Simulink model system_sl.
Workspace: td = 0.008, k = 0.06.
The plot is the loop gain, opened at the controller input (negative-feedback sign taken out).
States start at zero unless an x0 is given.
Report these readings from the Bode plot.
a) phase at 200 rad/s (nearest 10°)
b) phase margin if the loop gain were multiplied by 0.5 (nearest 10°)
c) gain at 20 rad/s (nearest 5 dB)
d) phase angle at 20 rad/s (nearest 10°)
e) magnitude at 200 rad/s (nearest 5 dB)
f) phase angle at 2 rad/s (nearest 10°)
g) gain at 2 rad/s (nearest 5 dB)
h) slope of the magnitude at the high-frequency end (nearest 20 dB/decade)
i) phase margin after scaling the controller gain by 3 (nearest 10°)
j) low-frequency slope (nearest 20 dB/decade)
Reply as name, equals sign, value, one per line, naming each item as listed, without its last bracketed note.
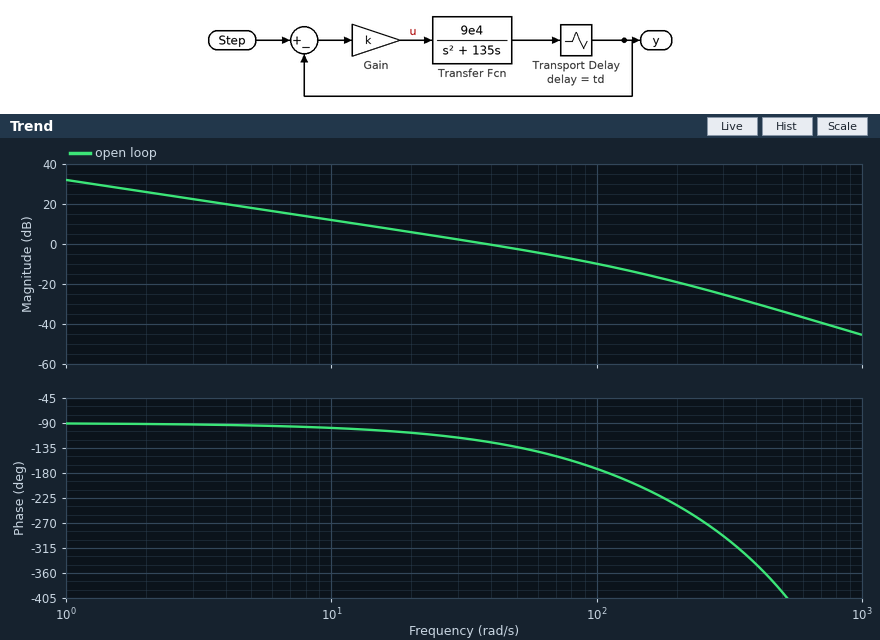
phase at 200 rad/s = -240°
phase margin if the loop gain were multiplied by 0.5 = 70°
gain at 20 rad/s = 5 dB
phase angle at 20 rad/s = -110°
magnitude at 200 rad/s = -20 dB
phase angle at 2 rad/s = -90°
gain at 2 rad/s = 25 dB
slope of the magnitude at the high-frequency end = -40 dB/decade
phase margin after scaling the controller gain by 3 = 10°
low-frequency slope = -20 dB/decade
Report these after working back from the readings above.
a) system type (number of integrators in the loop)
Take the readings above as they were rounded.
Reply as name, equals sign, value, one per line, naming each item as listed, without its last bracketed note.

system type = 1
